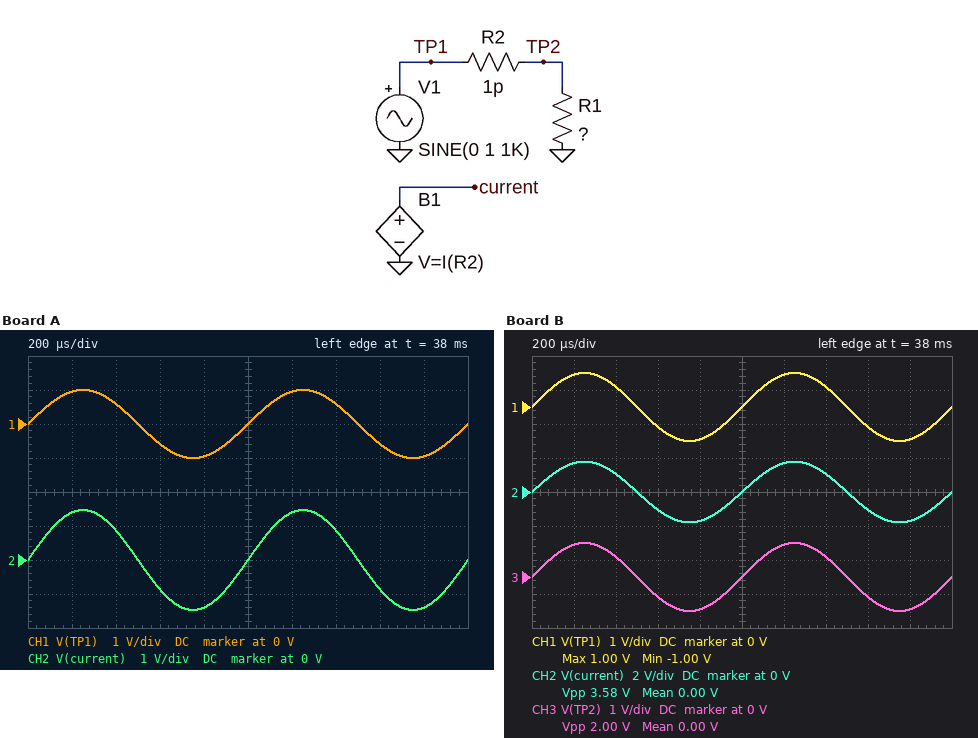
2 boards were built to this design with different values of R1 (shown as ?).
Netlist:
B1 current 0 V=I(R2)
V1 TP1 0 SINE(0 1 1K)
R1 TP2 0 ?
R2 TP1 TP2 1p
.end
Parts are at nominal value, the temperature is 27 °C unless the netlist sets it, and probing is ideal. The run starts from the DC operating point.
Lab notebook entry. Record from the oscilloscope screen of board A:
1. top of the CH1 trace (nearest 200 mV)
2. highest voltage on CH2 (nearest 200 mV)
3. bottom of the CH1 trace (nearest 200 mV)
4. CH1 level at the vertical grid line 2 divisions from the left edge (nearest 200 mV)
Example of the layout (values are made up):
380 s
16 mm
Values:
1.0 V
1.4 V
-1.0 V
600 mV
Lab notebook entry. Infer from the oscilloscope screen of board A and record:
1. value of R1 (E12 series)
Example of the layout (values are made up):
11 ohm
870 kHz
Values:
0.68 Ω
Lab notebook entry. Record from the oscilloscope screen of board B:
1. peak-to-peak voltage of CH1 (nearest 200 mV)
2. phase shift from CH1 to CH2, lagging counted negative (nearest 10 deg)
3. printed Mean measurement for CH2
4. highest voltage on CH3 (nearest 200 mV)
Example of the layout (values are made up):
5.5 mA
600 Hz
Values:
2.0 V
0 deg
0.00 V
1.0 V
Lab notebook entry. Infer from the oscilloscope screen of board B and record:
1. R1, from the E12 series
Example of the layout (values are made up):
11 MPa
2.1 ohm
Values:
0.56 Ω
